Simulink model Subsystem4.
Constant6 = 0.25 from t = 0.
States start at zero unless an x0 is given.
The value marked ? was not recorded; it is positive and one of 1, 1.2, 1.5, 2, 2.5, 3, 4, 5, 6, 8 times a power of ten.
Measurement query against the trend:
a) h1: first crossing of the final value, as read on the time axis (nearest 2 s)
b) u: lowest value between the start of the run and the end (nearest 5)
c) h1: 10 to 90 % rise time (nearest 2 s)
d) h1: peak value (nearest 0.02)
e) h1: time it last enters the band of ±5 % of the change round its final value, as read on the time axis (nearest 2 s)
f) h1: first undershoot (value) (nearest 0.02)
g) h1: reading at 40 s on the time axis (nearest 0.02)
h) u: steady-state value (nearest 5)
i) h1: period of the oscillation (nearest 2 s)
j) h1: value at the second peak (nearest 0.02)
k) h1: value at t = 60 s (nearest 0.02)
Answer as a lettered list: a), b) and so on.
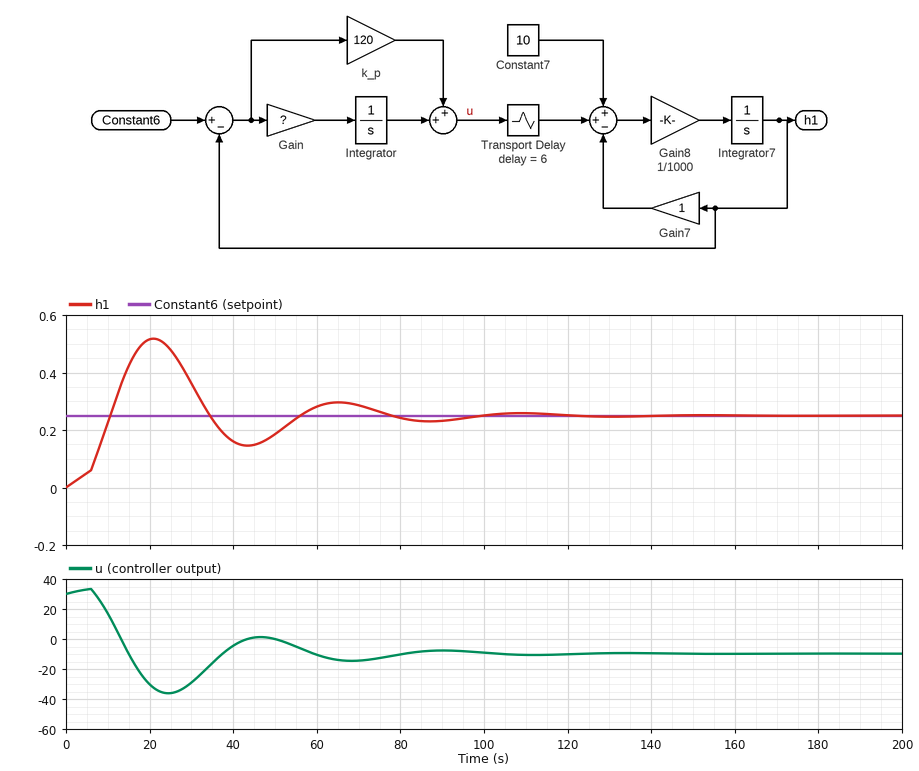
a) 10 s
b) -35
c) 8 s
d) 0.52
e) 94 s
f) 0.14
g) 0.16
h) -10
i) 44 s
j) 0.30
k) 0.28
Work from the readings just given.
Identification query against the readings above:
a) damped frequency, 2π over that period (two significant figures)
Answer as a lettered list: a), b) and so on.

a) 0.14 rad/s
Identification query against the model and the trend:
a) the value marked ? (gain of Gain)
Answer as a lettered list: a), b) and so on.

a) 8
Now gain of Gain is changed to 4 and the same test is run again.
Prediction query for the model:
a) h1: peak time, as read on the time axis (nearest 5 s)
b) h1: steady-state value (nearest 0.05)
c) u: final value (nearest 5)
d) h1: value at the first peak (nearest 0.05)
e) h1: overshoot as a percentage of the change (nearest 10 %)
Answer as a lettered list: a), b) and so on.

a) 20 s
b) 0.25
c) -10
d) 0.45
e) 80 %
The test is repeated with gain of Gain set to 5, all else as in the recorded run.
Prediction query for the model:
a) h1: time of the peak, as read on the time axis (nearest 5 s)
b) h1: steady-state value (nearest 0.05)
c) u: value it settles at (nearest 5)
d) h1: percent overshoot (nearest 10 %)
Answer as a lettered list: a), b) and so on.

a) 20 s
b) 0.25
c) -10
d) 90 %
